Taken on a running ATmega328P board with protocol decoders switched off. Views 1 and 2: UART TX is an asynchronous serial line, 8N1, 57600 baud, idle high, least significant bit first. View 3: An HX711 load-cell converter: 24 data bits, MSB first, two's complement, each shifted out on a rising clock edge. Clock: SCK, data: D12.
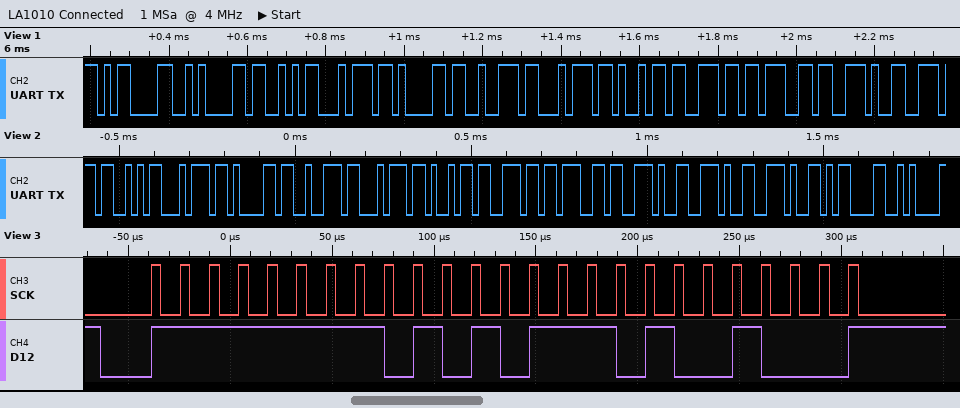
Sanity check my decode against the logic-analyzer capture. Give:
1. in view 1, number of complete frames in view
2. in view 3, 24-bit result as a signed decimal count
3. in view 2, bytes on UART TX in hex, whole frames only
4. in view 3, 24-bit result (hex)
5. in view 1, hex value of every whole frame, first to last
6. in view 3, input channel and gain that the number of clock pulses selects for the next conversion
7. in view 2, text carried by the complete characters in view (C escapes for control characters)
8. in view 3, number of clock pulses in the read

11
-43192
0x53 0x74 0x61 0x72 0x74 0x69 0x6E 0x67 0x2E 0x2E 0x2E 0x0D 0x0A
0xFF5748
0x0D 0x0A 0x53 0x74 0x61 0x72 0x74 0x69 0x6E 0x67 0x2E
channel A, gain 128
"Starting...\r\n"
25
